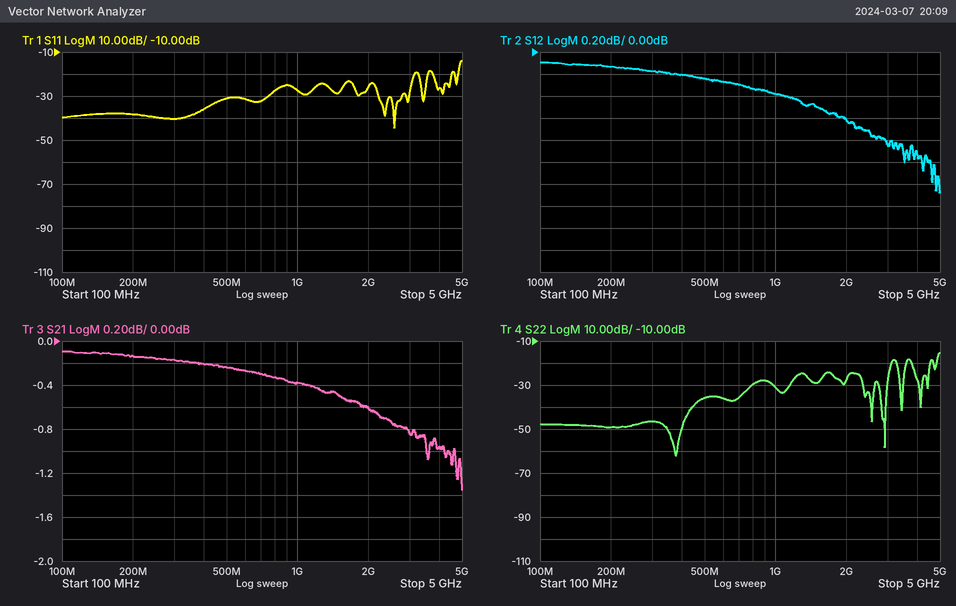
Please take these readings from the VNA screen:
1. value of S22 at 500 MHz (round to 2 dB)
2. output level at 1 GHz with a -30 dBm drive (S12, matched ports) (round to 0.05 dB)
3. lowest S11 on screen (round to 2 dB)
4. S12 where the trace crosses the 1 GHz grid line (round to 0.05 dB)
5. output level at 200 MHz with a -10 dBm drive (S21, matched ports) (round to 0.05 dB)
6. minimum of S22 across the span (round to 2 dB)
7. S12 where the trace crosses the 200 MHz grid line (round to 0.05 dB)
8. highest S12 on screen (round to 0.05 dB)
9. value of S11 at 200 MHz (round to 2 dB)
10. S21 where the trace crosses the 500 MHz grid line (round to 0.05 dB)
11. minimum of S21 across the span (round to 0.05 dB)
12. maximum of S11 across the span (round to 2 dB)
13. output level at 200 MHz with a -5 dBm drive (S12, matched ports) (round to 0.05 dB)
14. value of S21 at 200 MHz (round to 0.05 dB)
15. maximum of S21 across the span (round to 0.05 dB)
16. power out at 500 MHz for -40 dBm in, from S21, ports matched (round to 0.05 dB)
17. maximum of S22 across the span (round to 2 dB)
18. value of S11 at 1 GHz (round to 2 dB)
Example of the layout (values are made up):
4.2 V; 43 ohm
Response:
-36 dB; -30.40 dBm; -44 dB; -0.40 dB; -10.15 dBm; -62 dB; -0.15 dB; -0.10 dB; -38 dB; -0.25 dB; -1.35 dB; -14 dB; -5.15 dBm; -0.15 dB; -0.10 dB; -40.25 dBm; -16 dB; -28 dB
